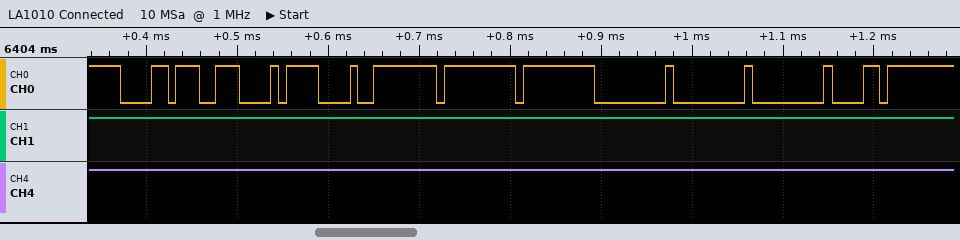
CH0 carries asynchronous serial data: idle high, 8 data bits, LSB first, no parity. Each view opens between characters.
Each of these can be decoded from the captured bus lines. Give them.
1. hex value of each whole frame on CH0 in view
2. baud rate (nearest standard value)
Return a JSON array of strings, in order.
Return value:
["D8, 0E, 0F, FE, FF, FF, 00, 00, 00, D8", "115200 baud"]
